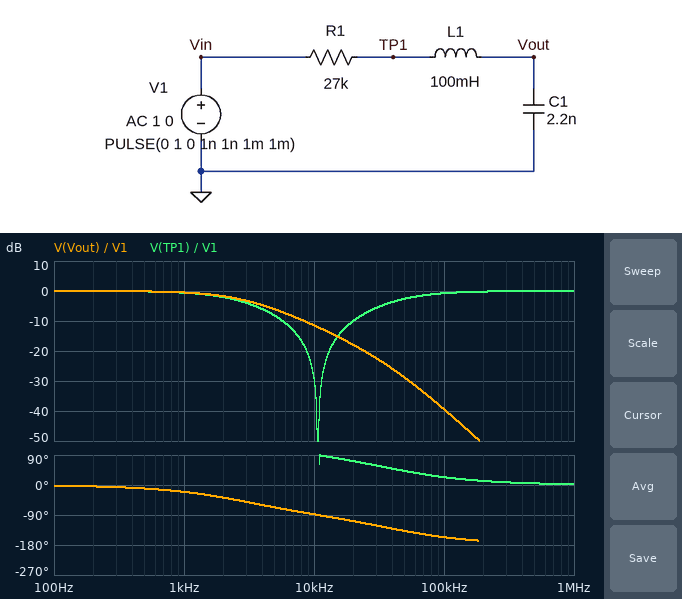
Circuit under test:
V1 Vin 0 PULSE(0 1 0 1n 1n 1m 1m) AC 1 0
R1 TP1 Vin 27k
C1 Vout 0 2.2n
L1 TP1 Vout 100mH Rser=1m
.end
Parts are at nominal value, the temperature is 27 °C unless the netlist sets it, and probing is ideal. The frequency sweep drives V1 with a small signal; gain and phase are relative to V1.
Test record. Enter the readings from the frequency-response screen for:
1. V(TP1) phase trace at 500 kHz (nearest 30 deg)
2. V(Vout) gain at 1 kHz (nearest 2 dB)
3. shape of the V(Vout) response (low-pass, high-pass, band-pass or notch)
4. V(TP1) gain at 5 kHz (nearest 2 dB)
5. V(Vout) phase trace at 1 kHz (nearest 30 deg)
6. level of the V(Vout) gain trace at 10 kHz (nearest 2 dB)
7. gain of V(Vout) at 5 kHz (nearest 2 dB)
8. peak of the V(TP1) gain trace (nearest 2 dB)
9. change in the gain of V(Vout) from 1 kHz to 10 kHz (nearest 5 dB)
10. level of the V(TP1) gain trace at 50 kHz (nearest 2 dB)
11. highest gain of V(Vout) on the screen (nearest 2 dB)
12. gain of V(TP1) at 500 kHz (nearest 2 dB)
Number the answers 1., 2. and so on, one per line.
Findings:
1. 0 deg
2. 0 dB
3. low-pass
4. -8 dB
5. -30 deg
6. -12 dB
7. -6 dB
8. 0 dB
9. -10 dB
10. -2 dB
11. 0 dB
12. 0 dB
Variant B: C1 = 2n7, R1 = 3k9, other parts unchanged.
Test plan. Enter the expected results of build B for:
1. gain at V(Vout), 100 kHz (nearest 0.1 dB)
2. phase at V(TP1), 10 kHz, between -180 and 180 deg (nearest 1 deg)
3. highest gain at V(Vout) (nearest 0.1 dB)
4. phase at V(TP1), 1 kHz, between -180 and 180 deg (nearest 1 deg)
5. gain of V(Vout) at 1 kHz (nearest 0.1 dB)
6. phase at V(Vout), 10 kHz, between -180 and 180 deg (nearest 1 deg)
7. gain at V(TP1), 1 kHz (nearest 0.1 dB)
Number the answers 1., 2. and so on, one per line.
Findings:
1. -40.5 dB
2. 84 deg
3. 4.3 dB
4. -4 deg
5. 0.1 dB
6. -96 deg
7. 0 dB
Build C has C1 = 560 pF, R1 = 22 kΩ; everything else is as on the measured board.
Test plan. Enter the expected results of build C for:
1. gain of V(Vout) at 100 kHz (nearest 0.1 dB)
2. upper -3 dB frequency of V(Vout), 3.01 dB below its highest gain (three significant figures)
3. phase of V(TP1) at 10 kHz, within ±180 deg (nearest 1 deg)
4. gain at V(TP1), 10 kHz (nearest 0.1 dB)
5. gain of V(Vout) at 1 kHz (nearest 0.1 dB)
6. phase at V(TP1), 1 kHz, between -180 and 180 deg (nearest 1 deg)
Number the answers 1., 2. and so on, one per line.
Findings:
1. -27.0 dB
2. 17.9 kHz
3. -45 deg
4. -3.0 dB
5. 0 dB
6. -4 deg
